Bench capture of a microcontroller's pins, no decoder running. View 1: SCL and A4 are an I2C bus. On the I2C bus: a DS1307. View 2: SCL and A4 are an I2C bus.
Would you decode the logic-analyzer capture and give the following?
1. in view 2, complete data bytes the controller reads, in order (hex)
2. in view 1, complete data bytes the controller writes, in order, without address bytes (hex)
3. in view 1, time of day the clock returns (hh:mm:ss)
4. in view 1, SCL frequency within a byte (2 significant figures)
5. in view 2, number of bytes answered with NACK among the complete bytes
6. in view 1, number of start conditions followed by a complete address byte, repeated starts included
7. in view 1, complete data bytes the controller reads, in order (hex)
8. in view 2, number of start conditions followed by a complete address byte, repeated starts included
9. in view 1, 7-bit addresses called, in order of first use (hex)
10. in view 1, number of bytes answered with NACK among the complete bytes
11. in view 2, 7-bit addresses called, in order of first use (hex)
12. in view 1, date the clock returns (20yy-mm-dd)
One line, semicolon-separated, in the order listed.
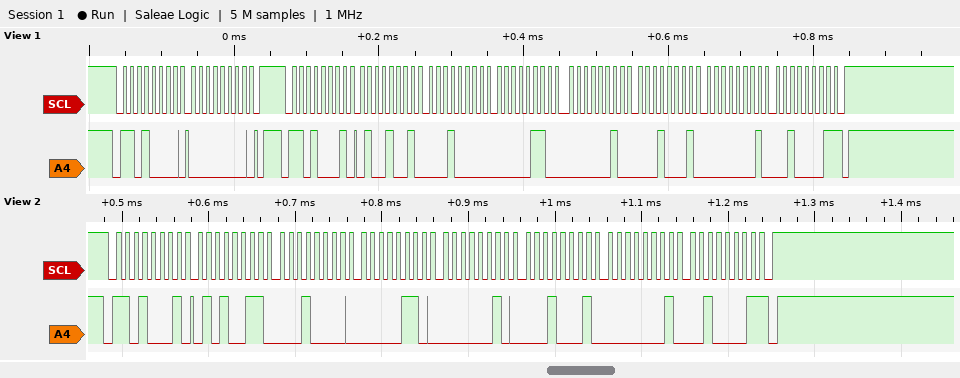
53 10 06 02 11 01 21; 00; 06:10:49; 100 kHz; 1; 2; 49 10 06 02 11 01 21; 1; 0x68; 1; 0x68; 2021-01-11
